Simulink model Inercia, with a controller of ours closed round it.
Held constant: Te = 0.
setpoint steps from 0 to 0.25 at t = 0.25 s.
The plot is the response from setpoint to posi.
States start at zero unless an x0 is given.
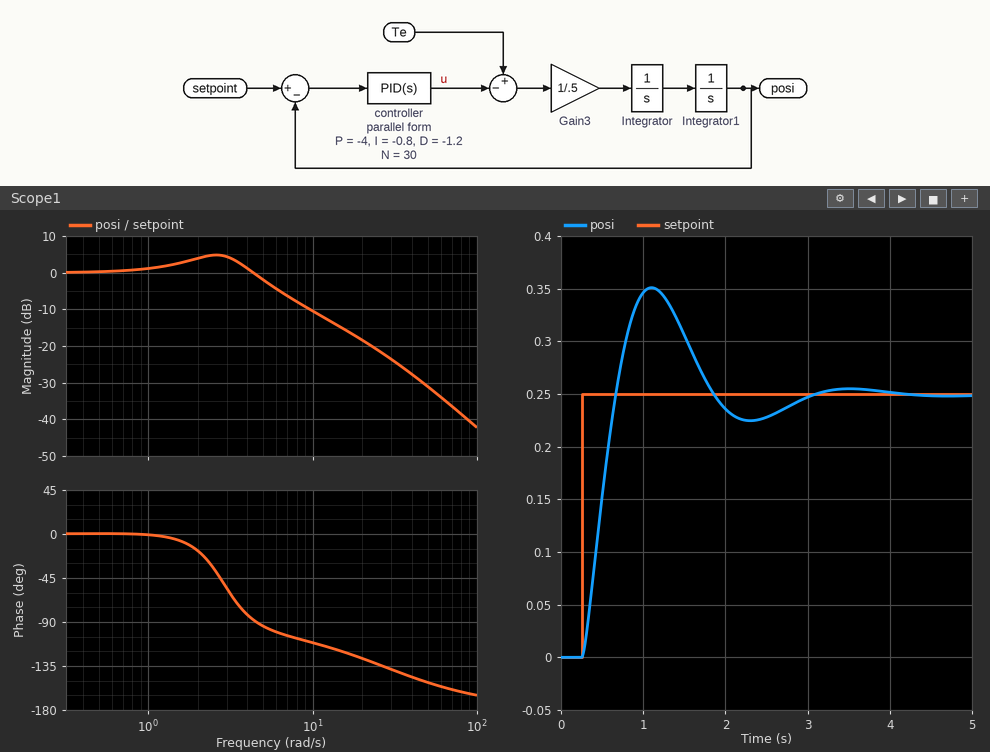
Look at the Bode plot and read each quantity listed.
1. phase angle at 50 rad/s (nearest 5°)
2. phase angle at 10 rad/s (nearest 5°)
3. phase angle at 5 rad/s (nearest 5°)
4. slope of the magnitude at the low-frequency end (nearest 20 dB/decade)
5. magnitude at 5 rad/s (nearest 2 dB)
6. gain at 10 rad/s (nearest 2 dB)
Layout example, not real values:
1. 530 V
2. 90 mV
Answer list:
1. -150°
2. -110°
3. -95°
4. 0 dB/decade
5. -2 dB
6. -10 dB
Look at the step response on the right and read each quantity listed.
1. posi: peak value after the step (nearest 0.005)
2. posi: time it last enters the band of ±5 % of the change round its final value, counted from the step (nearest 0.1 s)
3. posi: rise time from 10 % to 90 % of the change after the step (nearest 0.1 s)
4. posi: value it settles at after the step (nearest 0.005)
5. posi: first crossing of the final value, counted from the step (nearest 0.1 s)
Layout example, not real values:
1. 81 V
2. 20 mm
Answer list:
1. 0.350
2. 2.5 s
3. 0.3 s
4. 0.250
5. 0.4 s
